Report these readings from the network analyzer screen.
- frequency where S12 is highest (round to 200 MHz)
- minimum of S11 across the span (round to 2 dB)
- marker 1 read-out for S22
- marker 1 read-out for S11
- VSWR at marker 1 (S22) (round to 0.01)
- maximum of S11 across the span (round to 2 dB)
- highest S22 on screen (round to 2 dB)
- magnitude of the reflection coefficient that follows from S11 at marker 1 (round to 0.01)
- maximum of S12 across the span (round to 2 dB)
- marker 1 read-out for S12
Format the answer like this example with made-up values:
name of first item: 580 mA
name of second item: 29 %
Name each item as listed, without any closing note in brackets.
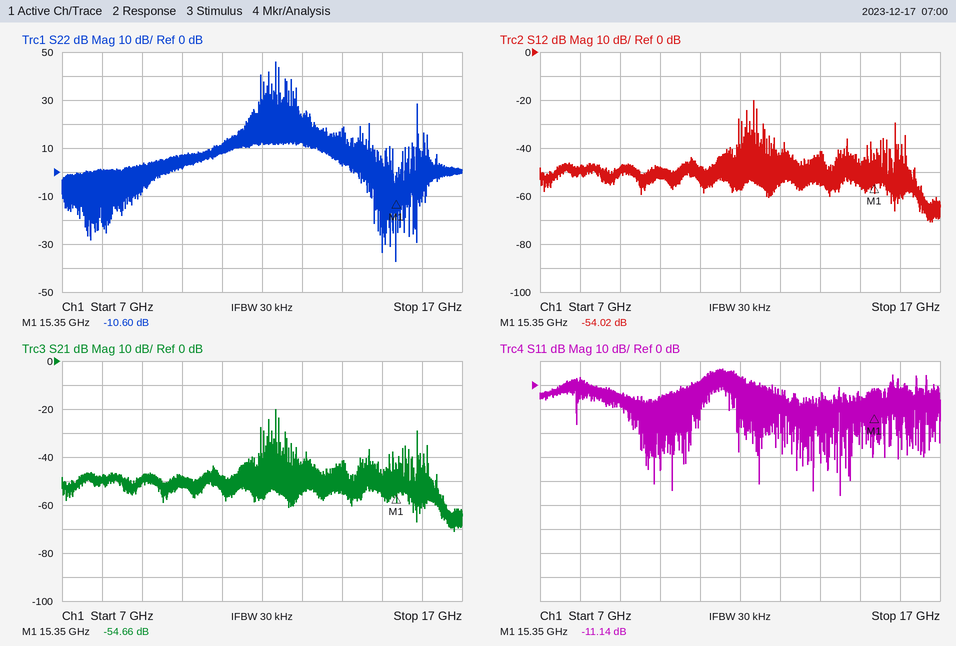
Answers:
frequency where S12 is highest: 12.4 GHz
minimum of S11 across the span: -46 dB
marker 1 read-out for S22: -10.60 dB
marker 1 read-out for S11: -11.14 dB
VSWR at marker 1 (S22): 1.84
maximum of S11 across the span: 6 dB
highest S22 on screen: 46 dB
magnitude of the reflection coefficient that follows from S11 at marker 1: 0.28
maximum of S12 across the span: -20 dB
marker 1 read-out for S12: -54.02 dB
